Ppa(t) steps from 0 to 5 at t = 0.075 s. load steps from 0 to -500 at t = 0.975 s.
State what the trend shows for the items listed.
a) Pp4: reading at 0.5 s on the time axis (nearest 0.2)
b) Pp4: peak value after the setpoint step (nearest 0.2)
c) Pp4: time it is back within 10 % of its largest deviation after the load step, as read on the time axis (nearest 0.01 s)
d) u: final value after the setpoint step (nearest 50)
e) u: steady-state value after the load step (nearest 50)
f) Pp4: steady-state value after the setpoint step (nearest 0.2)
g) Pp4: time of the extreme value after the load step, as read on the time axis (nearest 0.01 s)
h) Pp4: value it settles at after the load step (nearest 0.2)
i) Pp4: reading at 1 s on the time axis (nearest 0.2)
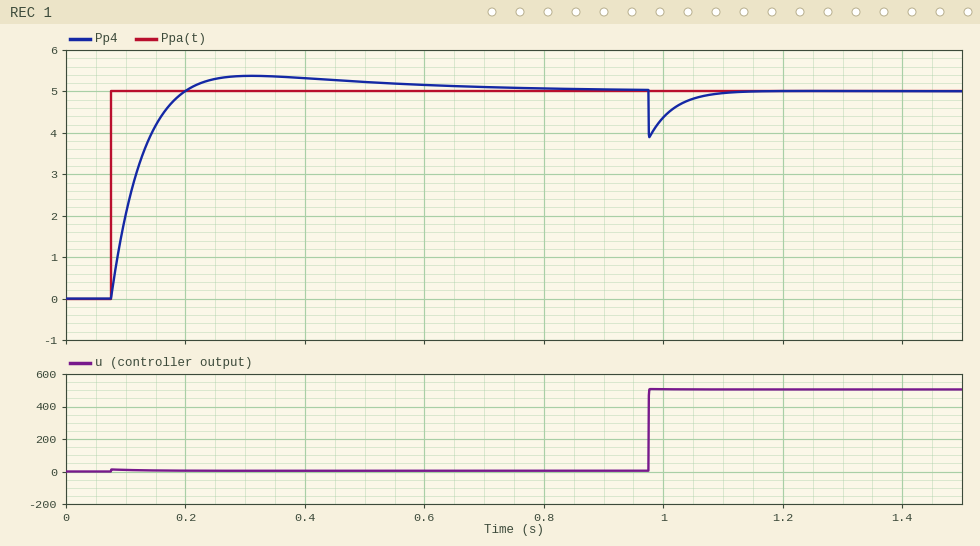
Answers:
5.2
5.4
1.07 s
0
500
5.0
0.98 s
5.0
4.4
